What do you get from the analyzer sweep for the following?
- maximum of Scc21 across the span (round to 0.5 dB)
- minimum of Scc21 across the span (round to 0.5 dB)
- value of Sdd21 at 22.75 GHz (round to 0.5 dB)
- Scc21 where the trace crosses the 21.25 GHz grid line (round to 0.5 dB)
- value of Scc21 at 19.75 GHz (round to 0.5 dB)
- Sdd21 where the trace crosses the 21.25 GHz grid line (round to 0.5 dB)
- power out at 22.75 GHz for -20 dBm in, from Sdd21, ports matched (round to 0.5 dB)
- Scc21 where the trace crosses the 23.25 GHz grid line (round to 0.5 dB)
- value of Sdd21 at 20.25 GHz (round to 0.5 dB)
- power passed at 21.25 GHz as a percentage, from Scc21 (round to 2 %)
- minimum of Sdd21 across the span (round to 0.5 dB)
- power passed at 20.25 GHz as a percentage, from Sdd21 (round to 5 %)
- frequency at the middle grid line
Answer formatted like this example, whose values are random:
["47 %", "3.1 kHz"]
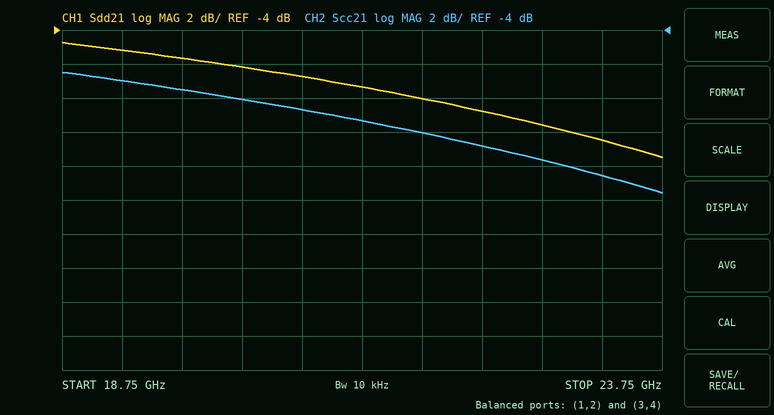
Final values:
["-6.5 dB", "-13.5 dB", "-9.5 dB", "-9.5 dB", "-7.5 dB", "-7.5 dB", "-29.5 dBm", "-12.5 dB", "-6.0 dB", "12 %", "-11.5 dB", "25 %", "21.25 GHz"]
